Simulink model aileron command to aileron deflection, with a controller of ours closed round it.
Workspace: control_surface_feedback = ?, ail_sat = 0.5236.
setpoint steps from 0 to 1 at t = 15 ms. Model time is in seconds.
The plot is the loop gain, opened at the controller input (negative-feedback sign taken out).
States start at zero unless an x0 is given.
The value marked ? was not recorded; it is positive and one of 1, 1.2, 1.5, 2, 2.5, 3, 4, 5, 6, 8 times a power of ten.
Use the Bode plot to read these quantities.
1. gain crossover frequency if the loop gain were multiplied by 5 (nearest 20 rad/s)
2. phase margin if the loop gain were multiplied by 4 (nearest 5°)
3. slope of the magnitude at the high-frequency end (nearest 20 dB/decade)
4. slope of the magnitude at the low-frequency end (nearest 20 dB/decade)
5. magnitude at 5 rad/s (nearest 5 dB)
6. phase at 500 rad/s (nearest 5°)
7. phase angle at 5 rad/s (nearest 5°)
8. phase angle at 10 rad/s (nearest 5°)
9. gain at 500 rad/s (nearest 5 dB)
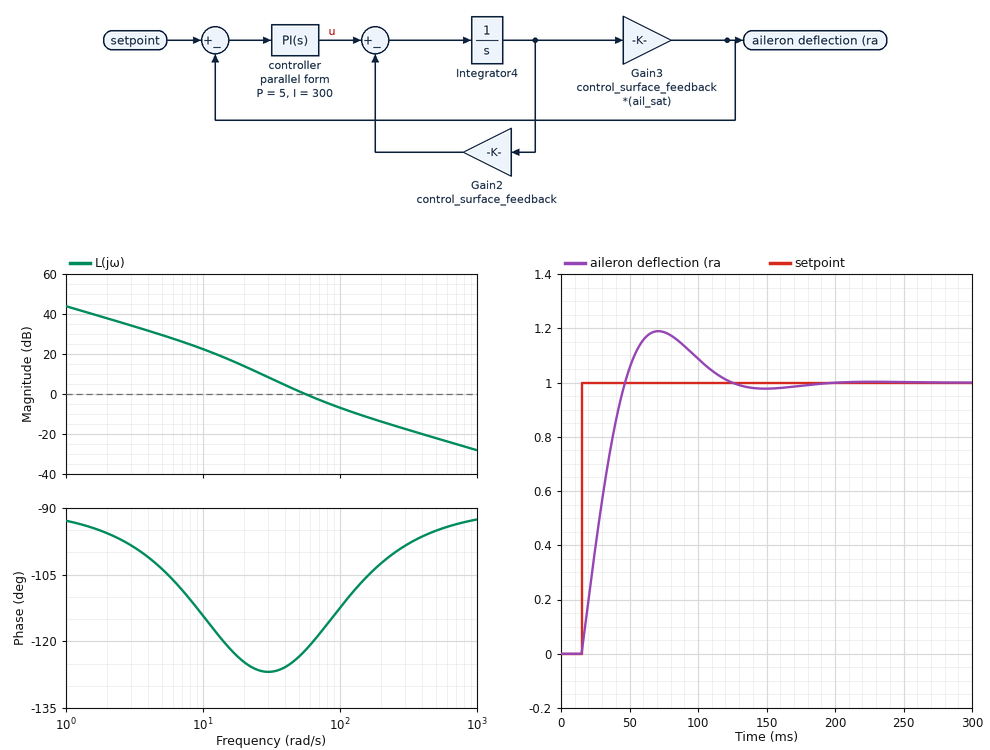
200 rad/s
75°
-20 dB/decade
-20 dB/decade
30 dB
-95°
-105°
-115°
-20 dB
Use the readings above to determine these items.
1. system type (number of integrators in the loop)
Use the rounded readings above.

1
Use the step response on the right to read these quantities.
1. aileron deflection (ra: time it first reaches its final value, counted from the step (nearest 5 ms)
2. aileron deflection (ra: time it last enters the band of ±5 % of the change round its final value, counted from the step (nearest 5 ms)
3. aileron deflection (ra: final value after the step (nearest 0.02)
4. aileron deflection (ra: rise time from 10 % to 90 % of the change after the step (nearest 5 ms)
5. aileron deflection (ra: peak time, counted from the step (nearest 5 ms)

30 ms
95 ms
1.00
25 ms
55 ms
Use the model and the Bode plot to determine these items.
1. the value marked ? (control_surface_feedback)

15
